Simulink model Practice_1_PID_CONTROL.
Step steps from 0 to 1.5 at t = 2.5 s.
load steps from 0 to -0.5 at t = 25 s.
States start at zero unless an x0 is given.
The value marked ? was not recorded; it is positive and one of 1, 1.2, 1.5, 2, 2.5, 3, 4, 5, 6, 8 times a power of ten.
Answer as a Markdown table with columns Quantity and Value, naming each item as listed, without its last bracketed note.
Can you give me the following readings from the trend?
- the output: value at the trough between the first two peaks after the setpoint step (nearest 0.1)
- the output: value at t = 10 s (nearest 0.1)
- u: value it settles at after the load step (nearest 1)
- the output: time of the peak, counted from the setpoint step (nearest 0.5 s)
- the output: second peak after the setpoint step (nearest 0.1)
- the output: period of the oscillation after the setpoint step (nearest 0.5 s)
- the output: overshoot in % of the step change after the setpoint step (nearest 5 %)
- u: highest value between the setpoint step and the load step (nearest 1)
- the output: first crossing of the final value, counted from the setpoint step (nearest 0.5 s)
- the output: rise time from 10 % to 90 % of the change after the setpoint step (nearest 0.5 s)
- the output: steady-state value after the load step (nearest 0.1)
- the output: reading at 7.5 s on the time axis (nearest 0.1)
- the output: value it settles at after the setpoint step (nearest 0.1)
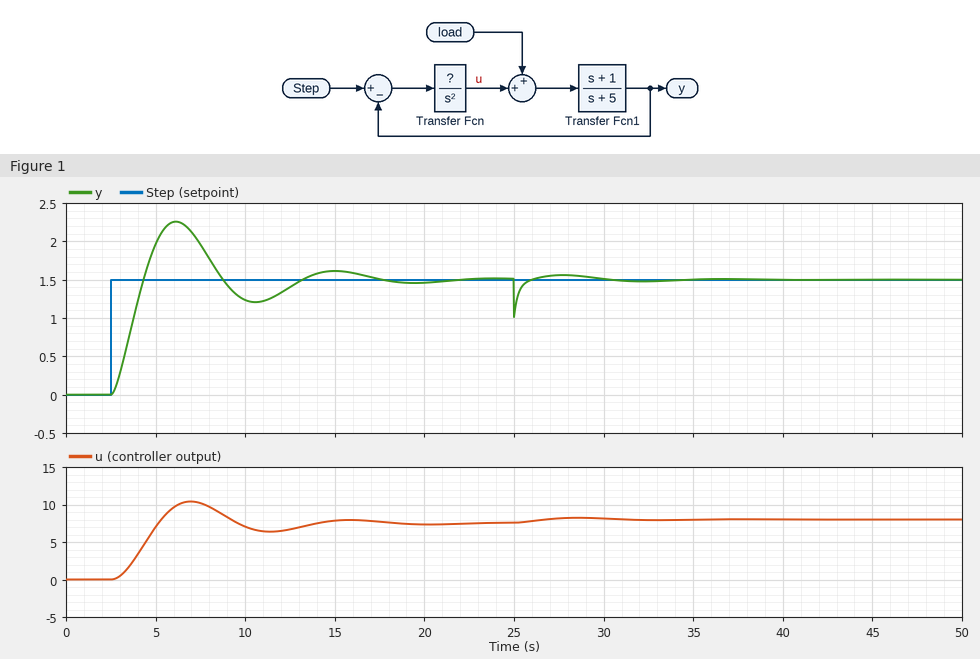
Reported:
| Quantity | Value |
|---|---|
| the output: value at the trough between the first two peaks after the setpoint step | 1.2 |
| the output: value at t = 10 s | 1.2 |
| u: value it settles at after the load step | 8 |
| the output: time of the peak, counted from the setpoint step | 3.5 s |
| the output: second peak after the setpoint step | 1.6 |
| the output: period of the oscillation after the setpoint step | 9.0 s |
| the output: overshoot in % of the step change after the setpoint step | 50 % |
| u: highest value between the setpoint step and the load step | 10 |
| the output: first crossing of the final value, counted from the setpoint step | 2.0 s |
| the output: rise time from 10 % to 90 % of the change after the setpoint step | 1.5 s |
| the output: steady-state value after the load step | 1.5 |
| the output: reading at 7.5 s on the time axis | 2.0 |
| the output: value it settles at after the setpoint step | 1.5 |
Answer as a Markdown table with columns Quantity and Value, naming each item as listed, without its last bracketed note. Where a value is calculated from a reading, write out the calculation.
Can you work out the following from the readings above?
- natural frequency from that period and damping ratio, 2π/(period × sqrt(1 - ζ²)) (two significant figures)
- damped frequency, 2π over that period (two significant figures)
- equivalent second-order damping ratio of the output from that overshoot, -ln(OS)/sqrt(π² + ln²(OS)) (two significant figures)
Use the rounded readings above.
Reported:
| Quantity | Value |
|---|---|
| natural frequency from that period and damping ratio, 2π/(period × sqrt(1 - ζ²)) | 2π / (9 × sqrt(1 - 0.22²)) = 0.72 rad/s |
| damped frequency, 2π over that period | 2π / 9 = 0.70 rad/s |
| equivalent second-order damping ratio of the output from that overshoot, -ln(OS)/sqrt(π² + ln²(OS)) | ln(0.5) = -0.693; 0.693 / sqrt(9.870 + 0.480) = 0.22 |
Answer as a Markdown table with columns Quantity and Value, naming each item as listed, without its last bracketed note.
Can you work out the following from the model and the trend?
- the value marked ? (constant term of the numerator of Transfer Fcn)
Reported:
| Quantity | Value |
|---|---|
| the value marked ? | 2.5 |
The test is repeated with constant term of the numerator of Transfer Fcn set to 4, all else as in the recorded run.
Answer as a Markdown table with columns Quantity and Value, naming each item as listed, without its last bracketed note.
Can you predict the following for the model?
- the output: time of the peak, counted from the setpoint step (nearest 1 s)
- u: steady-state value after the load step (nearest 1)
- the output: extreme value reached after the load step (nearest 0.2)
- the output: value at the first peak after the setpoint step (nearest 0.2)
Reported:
| Quantity | Value |
|---|---|
| the output: time of the peak, counted from the setpoint step | 3 s |
| u: steady-state value after the load step | 8 |
| the output: extreme value reached after the load step | 1.0 |
| the output: value at the first peak after the setpoint step | 2.2 |
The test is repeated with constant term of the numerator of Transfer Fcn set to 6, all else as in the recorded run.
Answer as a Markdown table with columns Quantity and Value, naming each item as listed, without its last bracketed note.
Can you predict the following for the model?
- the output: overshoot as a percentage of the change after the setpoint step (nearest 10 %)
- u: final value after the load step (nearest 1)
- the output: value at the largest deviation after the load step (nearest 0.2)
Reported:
| Quantity | Value |
|---|---|
| the output: overshoot as a percentage of the change after the setpoint step | 40 % |
| u: final value after the load step | 8 |
| the output: value at the largest deviation after the load step | 1.0 |
